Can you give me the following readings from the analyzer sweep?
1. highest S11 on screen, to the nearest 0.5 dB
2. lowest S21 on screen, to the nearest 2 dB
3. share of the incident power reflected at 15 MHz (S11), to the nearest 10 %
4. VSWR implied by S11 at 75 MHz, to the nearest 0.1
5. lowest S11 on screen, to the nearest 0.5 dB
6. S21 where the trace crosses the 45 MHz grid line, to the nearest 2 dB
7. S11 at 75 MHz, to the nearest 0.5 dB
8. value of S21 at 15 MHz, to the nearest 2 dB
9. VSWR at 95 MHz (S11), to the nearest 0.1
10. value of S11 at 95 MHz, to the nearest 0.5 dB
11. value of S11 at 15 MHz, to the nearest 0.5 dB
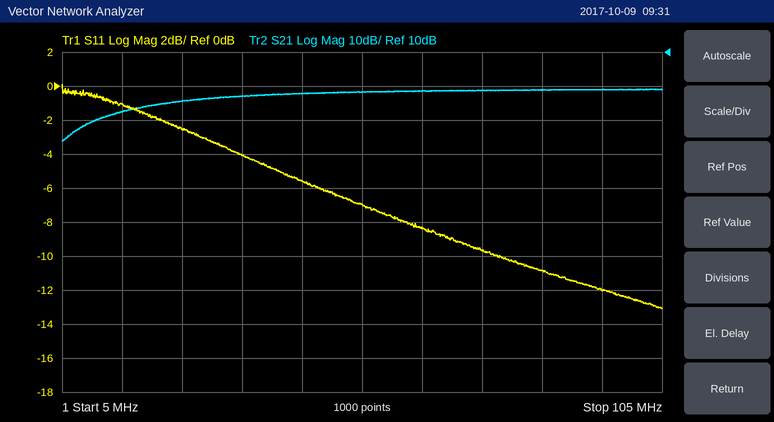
0.0 dB
-16 dB
80 %
2.0
-13.0 dB
-2 dB
-9.5 dB
-8 dB
1.7
-12.0 dB
-1.0 dB
